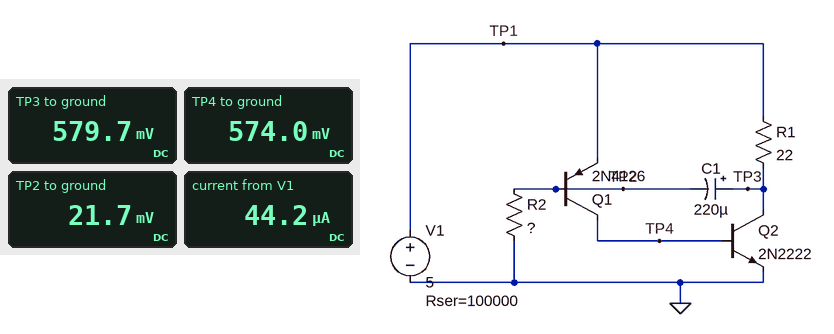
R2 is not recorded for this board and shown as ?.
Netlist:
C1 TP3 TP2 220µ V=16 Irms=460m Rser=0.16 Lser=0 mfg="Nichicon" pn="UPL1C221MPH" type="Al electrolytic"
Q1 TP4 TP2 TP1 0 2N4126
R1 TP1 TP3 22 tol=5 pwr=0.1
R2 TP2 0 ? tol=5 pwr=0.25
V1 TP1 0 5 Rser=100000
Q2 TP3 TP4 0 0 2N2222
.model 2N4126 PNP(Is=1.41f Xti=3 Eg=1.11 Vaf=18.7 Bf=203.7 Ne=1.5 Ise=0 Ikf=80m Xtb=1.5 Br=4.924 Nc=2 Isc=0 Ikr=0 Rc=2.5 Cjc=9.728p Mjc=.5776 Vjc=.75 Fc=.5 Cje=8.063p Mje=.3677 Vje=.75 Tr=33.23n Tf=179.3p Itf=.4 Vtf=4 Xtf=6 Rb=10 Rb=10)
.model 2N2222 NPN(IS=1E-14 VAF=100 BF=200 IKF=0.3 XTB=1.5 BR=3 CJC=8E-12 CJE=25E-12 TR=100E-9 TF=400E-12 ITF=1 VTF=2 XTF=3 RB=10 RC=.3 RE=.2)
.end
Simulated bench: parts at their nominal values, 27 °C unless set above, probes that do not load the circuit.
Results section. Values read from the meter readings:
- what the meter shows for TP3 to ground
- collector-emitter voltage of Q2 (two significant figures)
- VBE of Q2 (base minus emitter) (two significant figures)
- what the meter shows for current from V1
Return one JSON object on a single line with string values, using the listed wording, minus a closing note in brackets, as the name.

{"what the meter shows for TP3 to ground": "579.7 mV", "collector-emitter voltage of Q2": "580 mV", "VBE of Q2 (base minus emitter)": "570 mV", "what the meter shows for current from V1": "44.2 µA"}
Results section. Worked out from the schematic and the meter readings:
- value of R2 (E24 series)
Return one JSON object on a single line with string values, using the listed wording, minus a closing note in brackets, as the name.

{"value of R2": "39 kΩ"}
